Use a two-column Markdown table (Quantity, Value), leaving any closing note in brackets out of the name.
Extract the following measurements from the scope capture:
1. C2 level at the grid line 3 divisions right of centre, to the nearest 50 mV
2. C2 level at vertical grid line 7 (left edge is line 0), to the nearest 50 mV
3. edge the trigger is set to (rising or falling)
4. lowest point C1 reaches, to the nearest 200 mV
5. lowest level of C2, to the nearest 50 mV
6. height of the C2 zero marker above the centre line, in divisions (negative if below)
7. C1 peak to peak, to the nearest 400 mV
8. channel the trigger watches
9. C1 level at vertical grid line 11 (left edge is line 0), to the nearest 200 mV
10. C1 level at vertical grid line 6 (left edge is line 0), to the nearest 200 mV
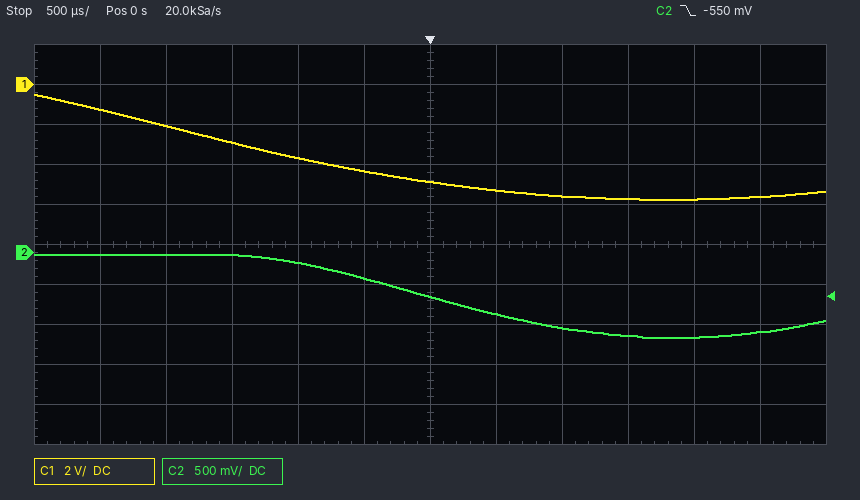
| Quantity | Value |
|---|---|
| C2 level at the grid line 3 divisions right of centre, to the nearest 50 mV | -1.05 V |
| C2 level at vertical grid line 7 (left edge is line 0), to the nearest 50 mV | -750 mV |
| edge the trigger is set to | falling |
| lowest point C1 reaches, to the nearest 200 mV | -5.8 V |
| lowest level of C2, to the nearest 50 mV | -1.05 V |
| height of the C2 zero marker above the centre line, in divisions | -0.2 div |
| C1 peak to peak, to the nearest 400 mV | 5.2 V |
| channel the trigger watches | C2 |
| C1 level at vertical grid line 11 (left edge is line 0), to the nearest 200 mV | -5.6 V |
| C1 level at vertical grid line 6 (left edge is line 0), to the nearest 200 mV | -4.8 V |
